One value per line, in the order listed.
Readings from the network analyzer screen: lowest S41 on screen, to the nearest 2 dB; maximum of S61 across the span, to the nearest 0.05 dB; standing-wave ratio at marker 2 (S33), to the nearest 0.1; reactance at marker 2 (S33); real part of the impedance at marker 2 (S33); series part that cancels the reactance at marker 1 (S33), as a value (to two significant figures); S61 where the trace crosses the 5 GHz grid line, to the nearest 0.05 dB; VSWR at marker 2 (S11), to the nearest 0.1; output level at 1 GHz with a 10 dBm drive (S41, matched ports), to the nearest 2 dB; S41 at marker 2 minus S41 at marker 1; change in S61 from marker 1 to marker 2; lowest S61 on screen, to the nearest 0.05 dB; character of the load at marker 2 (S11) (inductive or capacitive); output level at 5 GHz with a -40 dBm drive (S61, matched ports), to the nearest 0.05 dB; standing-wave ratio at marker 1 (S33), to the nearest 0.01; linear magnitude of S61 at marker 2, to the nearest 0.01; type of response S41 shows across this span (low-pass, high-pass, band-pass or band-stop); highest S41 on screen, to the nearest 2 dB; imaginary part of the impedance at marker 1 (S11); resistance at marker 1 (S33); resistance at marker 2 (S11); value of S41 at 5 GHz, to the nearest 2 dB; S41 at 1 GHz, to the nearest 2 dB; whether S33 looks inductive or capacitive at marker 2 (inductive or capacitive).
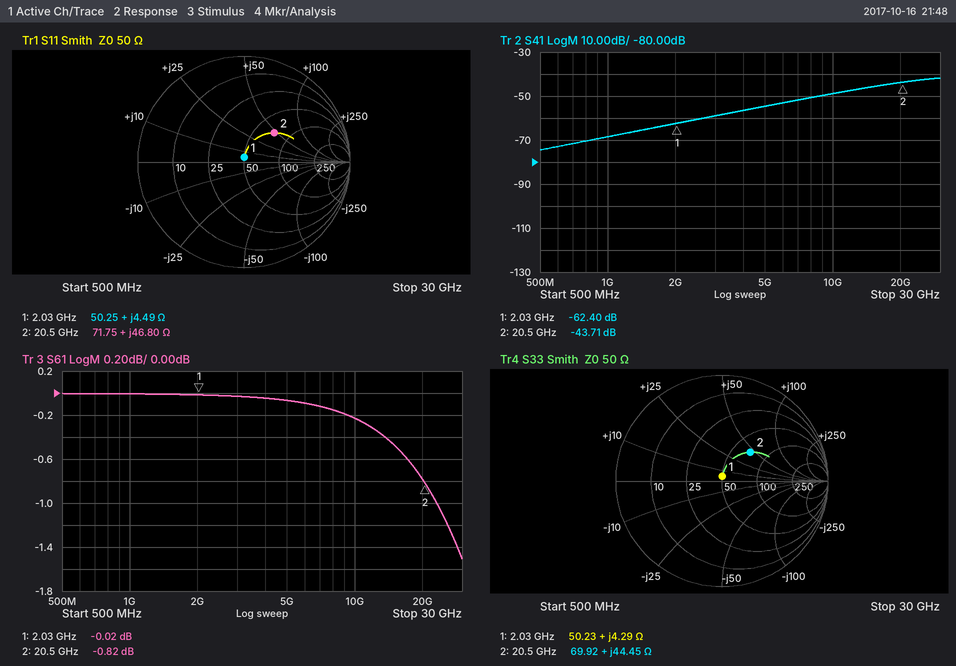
-74 dB
0.00 dB
2.2
+44.45 Ω
69.92 Ω
18 pF
-0.05 dB
2.3
-58 dBm
18.69 dB
-0.80 dB
-1.50 dB
inductive
-40.05 dBm
1.09
0.91
high-pass
-42 dB
+4.49 Ω
50.23 Ω
71.75 Ω
-54 dB
-68 dB
inductive
